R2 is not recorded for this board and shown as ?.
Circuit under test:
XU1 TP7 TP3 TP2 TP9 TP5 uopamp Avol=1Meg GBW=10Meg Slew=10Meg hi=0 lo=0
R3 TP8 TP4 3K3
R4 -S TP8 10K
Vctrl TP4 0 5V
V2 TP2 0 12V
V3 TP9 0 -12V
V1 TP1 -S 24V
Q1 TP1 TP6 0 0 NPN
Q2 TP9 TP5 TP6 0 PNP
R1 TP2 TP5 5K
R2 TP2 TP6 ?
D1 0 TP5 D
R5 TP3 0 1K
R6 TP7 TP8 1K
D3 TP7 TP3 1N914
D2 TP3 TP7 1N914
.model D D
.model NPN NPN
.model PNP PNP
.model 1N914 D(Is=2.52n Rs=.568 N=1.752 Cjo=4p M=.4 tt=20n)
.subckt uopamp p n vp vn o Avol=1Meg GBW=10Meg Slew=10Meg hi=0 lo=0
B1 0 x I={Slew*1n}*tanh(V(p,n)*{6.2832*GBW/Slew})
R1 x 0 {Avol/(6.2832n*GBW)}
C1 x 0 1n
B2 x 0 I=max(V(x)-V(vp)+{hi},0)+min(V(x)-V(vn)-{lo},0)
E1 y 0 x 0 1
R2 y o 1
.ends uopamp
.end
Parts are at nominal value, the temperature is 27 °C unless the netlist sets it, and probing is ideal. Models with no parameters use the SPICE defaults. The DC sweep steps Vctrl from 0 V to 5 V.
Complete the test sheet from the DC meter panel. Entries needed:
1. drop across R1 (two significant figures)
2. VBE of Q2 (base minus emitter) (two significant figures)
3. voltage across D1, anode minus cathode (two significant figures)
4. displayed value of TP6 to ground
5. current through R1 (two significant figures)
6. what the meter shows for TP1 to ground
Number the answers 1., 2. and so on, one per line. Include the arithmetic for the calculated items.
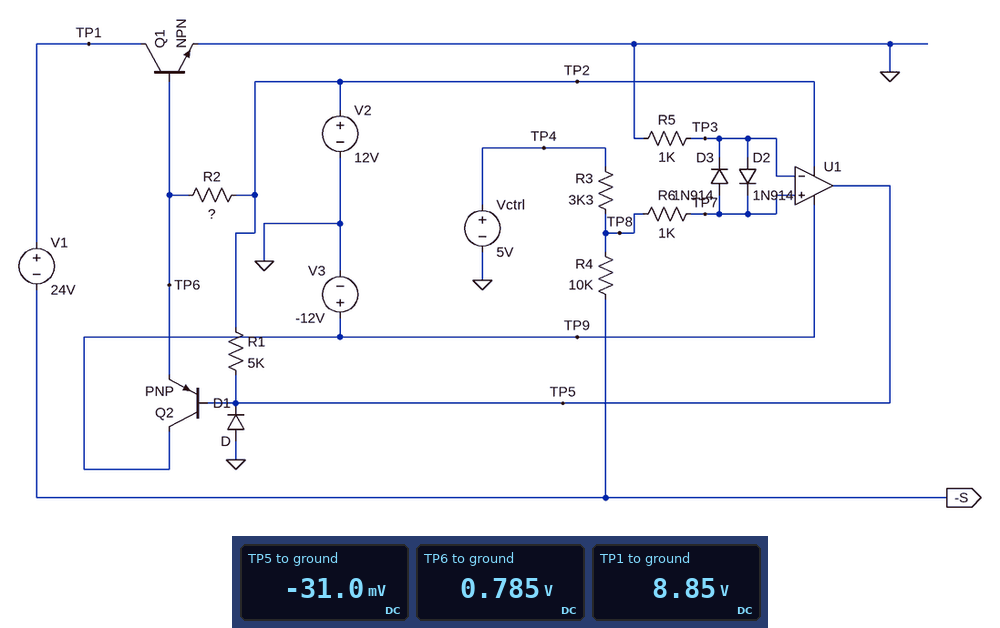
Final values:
1. 12 V - (-31 mV) = 12 V
2. -31 mV - 785 mV = -820 mV
3. 0 V - (-31 mV) = 31 mV
4. 0.785 V
5. (12 V - (-31 mV)) / 5 kΩ = 2.4 mA
6. 8.85 V
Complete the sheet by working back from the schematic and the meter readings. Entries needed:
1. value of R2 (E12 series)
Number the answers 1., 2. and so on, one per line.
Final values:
1. 2.2 kΩ
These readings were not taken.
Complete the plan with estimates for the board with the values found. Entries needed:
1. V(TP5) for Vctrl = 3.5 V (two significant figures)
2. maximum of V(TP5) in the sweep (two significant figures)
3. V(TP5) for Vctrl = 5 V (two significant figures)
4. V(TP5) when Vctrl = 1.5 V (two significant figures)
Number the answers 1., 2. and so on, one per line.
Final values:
1. -40 mV
2. -31 mV
3. -31 mV
4. -62 mV
